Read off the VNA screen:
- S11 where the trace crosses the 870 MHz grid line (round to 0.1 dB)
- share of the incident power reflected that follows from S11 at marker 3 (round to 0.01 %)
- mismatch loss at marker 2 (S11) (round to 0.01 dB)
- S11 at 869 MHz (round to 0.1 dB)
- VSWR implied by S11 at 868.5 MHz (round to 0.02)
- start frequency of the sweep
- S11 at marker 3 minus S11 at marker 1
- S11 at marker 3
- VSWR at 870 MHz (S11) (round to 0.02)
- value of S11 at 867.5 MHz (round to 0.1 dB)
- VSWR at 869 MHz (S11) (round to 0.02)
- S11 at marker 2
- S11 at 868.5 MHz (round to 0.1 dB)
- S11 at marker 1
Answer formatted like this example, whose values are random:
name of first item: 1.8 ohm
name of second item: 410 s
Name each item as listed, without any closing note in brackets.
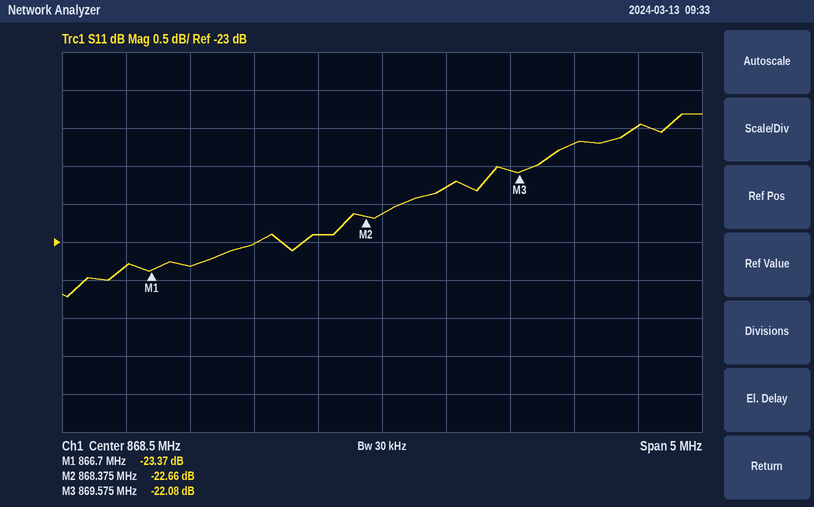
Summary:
S11 where the trace crosses the 870 MHz grid line: -21.7 dB
share of the incident power reflected that follows from S11 at marker 3: 0.62 %
mismatch loss at marker 2 (S11): 0.02 dB
S11 at 869 MHz: -22.3 dB
VSWR implied by S11 at 868.5 MHz: 1.16
start frequency of the sweep: 866 MHz
S11 at marker 3 minus S11 at marker 1: 1.29 dB
S11 at marker 3: -22.08 dB
VSWR at 870 MHz (S11): 1.18
value of S11 at 867.5 MHz: -23.0 dB
VSWR at 869 MHz (S11): 1.16
S11 at marker 2: -22.66 dB
S11 at 868.5 MHz: -22.6 dB
S11 at marker 1: -23.37 dB
